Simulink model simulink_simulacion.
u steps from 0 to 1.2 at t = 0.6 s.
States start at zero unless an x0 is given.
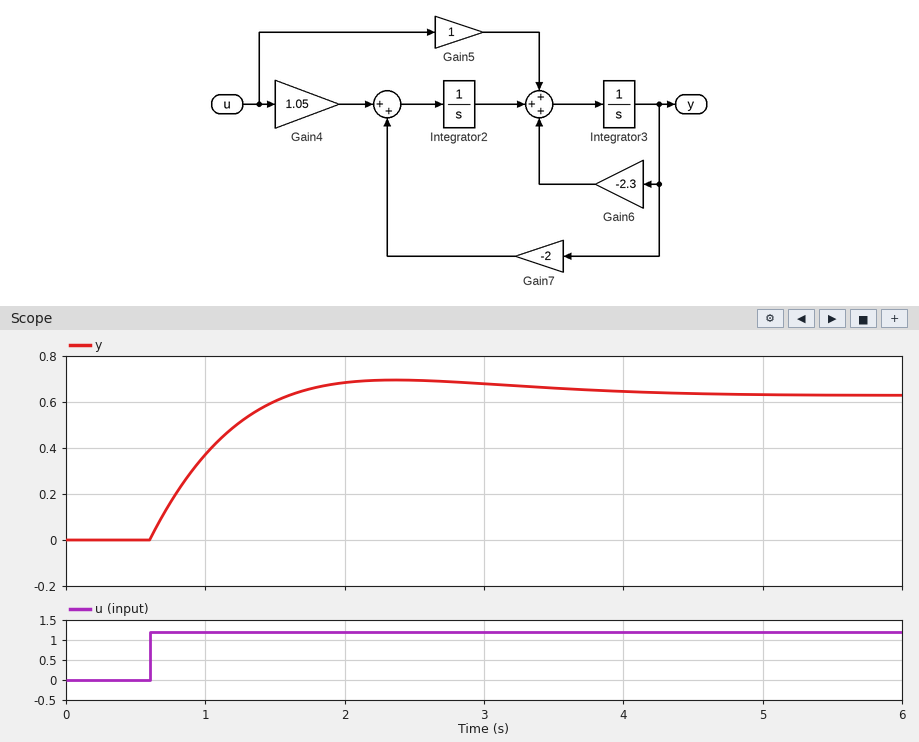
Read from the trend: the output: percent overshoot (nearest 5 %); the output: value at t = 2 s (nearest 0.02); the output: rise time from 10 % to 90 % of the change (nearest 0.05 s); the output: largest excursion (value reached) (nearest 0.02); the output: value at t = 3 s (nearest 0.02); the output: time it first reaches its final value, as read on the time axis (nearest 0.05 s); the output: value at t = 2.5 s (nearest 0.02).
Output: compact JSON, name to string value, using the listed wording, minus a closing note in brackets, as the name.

{"the output: percent overshoot": "10 %", "the output: value at t = 2 s": "0.68", "the output: rise time from 10 % to 90 % of the change": "0.75 s", "the output: largest excursion (value reached)": "0.70", "the output: value at t = 3 s": "0.68", "the output: time it first reaches its final value, as read on the time axis": "1.60 s", "the output: value at t = 2.5 s": "0.70"}
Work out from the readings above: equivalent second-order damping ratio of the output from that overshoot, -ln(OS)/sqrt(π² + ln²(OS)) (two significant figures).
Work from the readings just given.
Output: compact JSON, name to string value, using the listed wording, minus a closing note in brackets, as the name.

{"equivalent second-order damping ratio of the output from that overshoot, -ln(OS)/sqrt(π² + ln²(OS))": "0.59"}
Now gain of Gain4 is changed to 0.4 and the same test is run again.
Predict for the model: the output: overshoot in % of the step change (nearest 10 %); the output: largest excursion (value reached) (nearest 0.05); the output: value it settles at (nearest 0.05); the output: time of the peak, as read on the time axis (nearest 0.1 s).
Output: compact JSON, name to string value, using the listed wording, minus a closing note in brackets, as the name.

{"the output: overshoot in % of the step change": "90 %", "the output: largest excursion (value reached)": "0.45", "the output: value it settles at": "0.25", "the output: time of the peak, as read on the time axis": "1.6 s"}
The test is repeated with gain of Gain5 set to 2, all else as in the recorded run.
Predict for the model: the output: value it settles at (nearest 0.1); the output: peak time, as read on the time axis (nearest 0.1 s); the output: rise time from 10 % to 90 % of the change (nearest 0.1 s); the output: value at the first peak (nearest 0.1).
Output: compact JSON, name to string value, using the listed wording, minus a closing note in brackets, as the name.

{"the output: value it settles at": "0.6", "the output: peak time, as read on the time axis": "1.7 s", "the output: rise time from 10 % to 90 % of the change": "0.3 s", "the output: value at the first peak": "1.0"}
